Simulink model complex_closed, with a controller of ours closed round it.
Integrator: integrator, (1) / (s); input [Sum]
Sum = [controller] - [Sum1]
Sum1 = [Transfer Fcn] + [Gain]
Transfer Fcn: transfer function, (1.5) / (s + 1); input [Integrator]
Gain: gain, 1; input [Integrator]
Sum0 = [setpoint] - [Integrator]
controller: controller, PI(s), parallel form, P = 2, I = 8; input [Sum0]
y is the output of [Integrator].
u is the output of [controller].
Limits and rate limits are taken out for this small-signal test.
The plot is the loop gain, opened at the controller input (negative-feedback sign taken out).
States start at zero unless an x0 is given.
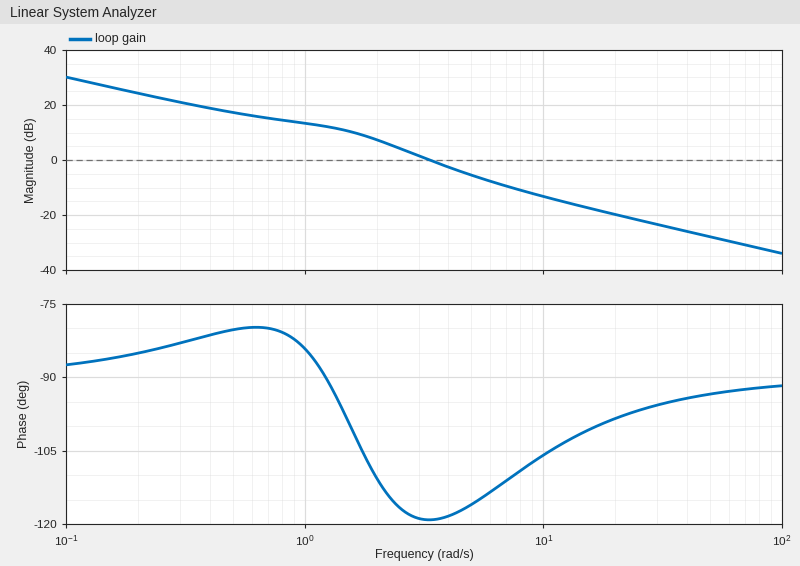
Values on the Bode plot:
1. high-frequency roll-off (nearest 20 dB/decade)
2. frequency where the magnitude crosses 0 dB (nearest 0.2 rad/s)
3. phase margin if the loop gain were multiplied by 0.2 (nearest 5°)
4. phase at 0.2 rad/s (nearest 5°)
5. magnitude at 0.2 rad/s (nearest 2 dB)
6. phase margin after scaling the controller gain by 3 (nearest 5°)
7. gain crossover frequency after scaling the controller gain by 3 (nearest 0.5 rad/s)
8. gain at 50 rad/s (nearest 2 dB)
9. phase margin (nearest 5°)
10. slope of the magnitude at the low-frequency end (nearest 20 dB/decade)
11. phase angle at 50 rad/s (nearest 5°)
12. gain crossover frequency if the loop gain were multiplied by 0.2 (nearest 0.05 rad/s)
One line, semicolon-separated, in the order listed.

-20 dB/decade; 3.4 rad/s; 100°; -85°; 24 dB; 70°; 7.0 rad/s; -28 dB; 60°; -20 dB/decade; -95°; 0.90 rad/s
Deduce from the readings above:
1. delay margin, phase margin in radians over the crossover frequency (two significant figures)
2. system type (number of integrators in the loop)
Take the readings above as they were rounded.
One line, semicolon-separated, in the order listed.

0.31 s; 1
